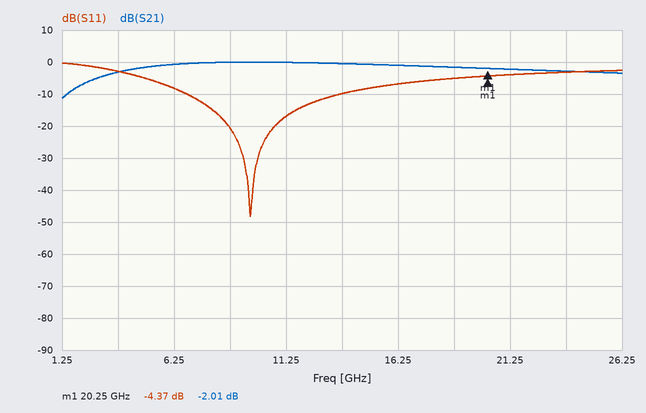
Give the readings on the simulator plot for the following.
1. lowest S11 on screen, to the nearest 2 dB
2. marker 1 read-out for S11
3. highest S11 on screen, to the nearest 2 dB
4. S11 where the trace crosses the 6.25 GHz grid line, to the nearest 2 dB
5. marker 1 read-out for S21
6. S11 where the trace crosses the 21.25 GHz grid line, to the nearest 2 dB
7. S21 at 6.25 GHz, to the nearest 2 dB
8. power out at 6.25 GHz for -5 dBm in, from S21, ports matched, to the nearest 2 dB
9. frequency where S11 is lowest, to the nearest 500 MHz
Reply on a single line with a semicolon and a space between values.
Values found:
-48 dB; -4.37 dB; 0 dB; -8 dB; -2.01 dB; -4 dB; 0 dB; -6 dBm; 9.5 GHz
